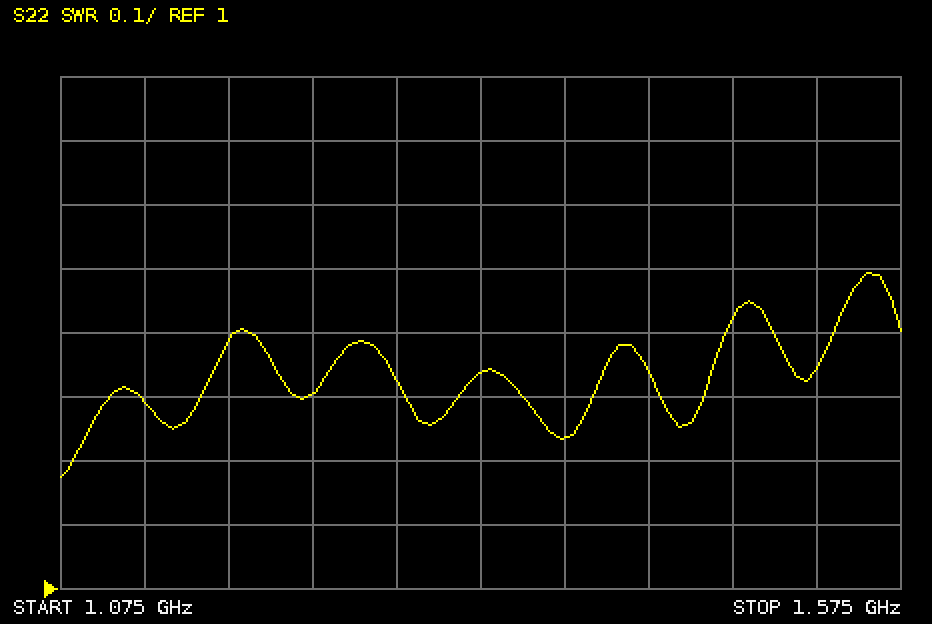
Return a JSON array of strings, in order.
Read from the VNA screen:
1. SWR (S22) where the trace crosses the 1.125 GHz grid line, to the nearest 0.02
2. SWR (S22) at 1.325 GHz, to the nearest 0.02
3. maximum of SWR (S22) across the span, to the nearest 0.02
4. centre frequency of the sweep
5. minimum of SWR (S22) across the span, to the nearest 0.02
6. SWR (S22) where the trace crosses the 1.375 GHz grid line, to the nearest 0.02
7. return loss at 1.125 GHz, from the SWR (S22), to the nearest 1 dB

["1.30", "1.34", "1.50", "1.325 GHz", "1.18", "1.24", "18 dB"]
